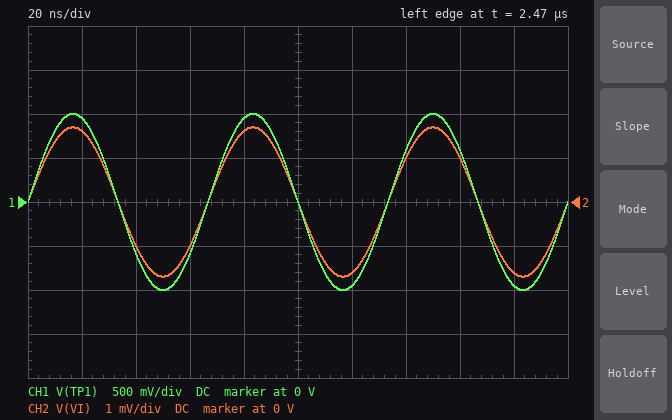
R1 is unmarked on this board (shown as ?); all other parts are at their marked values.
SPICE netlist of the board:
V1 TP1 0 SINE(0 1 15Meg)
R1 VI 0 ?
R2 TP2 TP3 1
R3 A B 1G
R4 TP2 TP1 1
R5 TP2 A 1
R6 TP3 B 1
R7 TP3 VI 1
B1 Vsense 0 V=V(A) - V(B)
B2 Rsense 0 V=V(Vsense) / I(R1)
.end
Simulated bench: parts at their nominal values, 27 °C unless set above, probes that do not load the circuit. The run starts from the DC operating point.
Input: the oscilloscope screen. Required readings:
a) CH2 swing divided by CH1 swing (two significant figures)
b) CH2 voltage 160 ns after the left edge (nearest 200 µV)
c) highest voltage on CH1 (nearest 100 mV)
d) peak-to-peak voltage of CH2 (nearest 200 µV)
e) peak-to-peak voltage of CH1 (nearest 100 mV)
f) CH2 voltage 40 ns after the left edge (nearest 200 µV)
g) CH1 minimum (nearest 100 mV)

0.0017
1.0 mV
1.0 V
3.4 mV
2.0 V
-1.0 mV
-1.0 V
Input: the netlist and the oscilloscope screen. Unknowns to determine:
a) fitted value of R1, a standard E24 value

5.1 mΩ
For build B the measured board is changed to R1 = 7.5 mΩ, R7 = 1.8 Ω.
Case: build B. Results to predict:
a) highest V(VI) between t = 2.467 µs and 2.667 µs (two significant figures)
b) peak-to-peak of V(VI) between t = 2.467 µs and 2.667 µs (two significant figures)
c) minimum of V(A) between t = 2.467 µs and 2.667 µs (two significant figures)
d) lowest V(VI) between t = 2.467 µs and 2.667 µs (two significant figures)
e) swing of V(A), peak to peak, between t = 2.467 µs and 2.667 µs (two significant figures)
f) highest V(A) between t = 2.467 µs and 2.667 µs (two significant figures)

2.0 mV
3.9 mV
-740 mV
-2.0 mV
1.5 V
740 mV
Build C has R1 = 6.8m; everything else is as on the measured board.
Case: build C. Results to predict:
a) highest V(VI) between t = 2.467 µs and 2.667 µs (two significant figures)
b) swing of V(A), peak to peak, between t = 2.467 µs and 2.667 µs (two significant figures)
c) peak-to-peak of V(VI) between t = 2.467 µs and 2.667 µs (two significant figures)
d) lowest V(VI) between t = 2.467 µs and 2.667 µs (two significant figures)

2.3 mV
1.3 V
4.5 mV
-2.3 mV
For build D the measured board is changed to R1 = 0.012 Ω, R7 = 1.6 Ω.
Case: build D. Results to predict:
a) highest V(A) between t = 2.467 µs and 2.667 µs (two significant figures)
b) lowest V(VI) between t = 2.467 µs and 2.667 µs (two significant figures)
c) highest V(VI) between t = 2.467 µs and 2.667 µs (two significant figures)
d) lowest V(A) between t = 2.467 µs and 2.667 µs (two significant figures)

720 mV
-3.3 mV
3.3 mV
-720 mV
